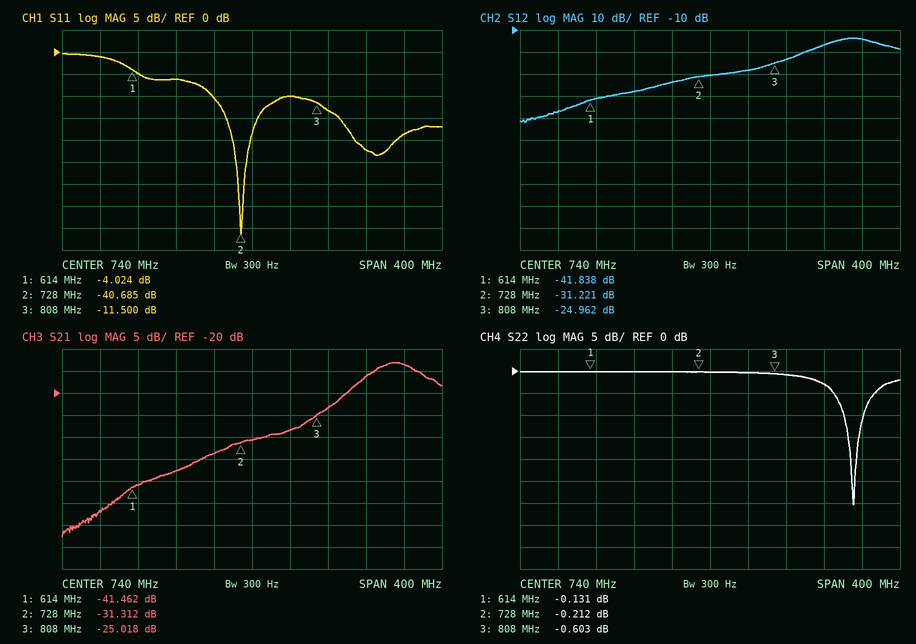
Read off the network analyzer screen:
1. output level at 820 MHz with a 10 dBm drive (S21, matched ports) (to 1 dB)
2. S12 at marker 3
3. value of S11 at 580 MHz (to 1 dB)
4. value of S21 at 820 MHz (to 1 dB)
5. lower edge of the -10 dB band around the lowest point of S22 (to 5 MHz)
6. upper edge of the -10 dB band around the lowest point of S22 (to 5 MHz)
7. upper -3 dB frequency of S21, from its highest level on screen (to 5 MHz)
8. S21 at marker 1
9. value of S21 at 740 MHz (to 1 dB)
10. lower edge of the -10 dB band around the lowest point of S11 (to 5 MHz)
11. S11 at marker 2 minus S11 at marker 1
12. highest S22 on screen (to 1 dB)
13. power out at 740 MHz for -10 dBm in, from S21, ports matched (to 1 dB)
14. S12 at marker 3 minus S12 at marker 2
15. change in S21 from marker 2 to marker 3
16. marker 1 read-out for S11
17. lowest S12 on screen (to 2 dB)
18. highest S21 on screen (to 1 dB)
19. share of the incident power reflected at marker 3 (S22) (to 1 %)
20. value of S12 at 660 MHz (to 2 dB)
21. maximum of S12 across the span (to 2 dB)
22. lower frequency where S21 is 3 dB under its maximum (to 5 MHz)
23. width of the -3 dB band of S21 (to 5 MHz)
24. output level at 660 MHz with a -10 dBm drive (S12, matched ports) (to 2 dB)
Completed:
-13 dBm
-24.962 dB
-1 dB
-23 dB
880 MHz
900 MHz
920 MHz
-41.462 dB
-31 dB
700 MHz
-36.661 dB
0 dB
-41 dBm
6.259 dB
6.294 dB
-4.024 dB
-52 dB
-13 dB
87 %
-38 dB
-14 dB
860 MHz
60 MHz
-48 dBm
